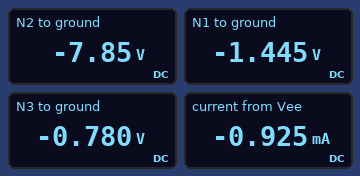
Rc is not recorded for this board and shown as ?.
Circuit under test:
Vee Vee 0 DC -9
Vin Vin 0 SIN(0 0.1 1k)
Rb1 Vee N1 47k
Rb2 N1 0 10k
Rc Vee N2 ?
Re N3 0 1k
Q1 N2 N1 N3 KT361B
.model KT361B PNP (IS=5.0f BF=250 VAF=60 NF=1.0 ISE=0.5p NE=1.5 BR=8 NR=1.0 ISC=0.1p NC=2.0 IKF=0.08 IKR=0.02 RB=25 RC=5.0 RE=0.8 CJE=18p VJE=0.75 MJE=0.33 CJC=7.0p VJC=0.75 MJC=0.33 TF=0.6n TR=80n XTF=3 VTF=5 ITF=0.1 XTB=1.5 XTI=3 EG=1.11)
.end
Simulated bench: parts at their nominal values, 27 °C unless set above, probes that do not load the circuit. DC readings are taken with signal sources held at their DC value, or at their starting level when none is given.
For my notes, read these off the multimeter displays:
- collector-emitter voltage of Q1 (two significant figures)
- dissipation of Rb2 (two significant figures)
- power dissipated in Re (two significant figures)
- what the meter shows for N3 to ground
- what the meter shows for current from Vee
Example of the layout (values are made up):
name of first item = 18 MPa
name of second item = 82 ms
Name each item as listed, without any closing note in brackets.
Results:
collector-emitter voltage of Q1 = -7.1 V
dissipation of Rb2 = 210 µW
power dissipated in Re = 610 µW
what the meter shows for N3 to ground = -0.780 V
what the meter shows for current from Vee = -0.925 mA
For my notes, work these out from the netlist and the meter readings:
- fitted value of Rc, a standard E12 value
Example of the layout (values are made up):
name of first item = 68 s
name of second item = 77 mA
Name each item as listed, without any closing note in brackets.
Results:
fitted value of Rc, a standard E12 value = 1.5 kΩ
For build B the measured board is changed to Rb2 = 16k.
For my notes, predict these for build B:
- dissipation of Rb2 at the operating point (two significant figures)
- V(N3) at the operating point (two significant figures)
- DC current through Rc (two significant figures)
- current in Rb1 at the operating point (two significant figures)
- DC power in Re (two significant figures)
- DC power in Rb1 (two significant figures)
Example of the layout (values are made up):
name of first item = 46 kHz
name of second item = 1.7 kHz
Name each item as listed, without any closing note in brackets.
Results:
dissipation of Rb2 at the operating point = 250 µW
V(N3) at the operating point = -1.3 V
DC current through Rc = 1.3 mA
current in Rb1 at the operating point = 150 µA
DC power in Re = 1.7 mW
DC power in Rb1 = 1.0 mW
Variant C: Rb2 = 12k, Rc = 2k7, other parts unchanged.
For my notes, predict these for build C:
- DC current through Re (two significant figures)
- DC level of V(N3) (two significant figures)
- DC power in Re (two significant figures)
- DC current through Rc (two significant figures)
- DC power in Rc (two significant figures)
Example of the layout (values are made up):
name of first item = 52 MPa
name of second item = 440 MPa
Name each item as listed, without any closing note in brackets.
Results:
DC current through Re = 970 µA
DC level of V(N3) = -970 mV
DC power in Re = 950 µW
DC current through Rc = 950 µA
DC power in Rc = 2.5 mW
